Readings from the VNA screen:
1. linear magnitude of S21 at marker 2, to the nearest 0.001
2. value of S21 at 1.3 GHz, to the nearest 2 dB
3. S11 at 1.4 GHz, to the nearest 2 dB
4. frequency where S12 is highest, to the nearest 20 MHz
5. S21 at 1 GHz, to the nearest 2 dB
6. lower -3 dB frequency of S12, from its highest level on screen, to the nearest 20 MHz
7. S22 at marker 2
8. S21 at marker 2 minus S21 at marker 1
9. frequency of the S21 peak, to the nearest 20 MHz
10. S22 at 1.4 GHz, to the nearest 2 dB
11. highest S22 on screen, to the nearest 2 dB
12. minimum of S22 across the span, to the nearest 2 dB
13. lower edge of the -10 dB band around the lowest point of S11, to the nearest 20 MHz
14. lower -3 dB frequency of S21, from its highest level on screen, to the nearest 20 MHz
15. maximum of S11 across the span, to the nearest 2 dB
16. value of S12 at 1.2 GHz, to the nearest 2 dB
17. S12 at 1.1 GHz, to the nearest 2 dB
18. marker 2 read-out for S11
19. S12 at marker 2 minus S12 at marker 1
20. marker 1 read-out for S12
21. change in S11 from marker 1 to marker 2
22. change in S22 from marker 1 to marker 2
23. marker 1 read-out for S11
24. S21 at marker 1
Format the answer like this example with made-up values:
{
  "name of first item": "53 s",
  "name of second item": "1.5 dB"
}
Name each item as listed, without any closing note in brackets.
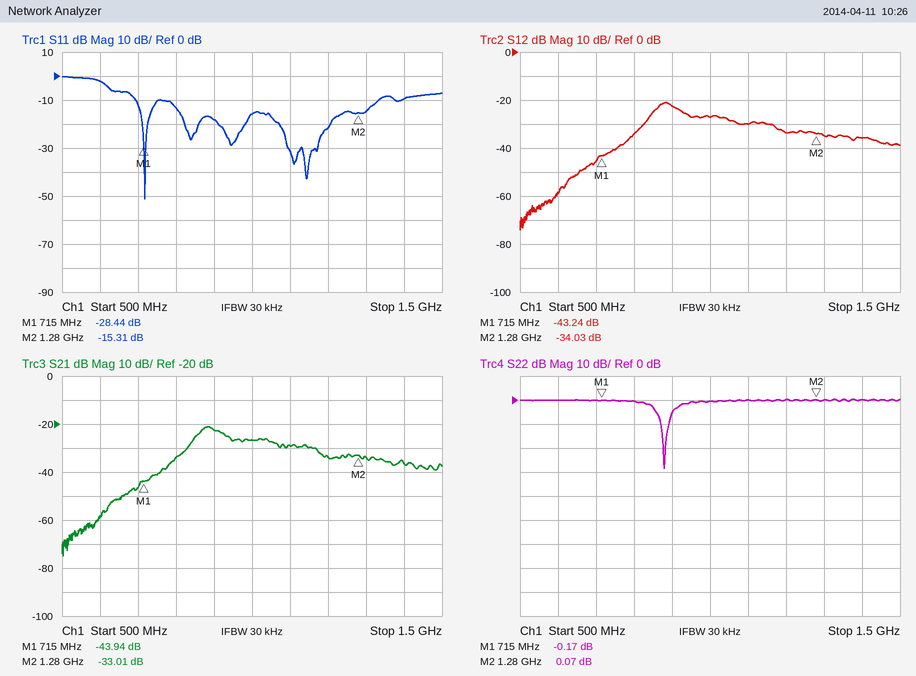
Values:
{
  "linear magnitude of S21 at marker 2, to the nearest 0.001": "0.022",
  "value of S21 at 1.3 GHz, to the nearest 2 dB": "-34 dB",
  "S11 at 1.4 GHz, to the nearest 2 dB": "-10 dB",
  "frequency where S12 is highest, to the nearest 20 MHz": "880 MHz",
  "S21 at 1 GHz, to the nearest 2 dB": "-26 dB",
  "lower -3 dB frequency of S12, from its highest level on screen, to the nearest 20 MHz": "860 MHz",
  "S22 at marker 2": "0.07 dB",
  "S21 at marker 2 minus S21 at marker 1": "10.93 dB",
  "frequency of the S21 peak, to the nearest 20 MHz": "880 MHz",
  "S22 at 1.4 GHz, to the nearest 2 dB": "0 dB",
  "highest S22 on screen, to the nearest 2 dB": "0 dB",
  "minimum of S22 across the span, to the nearest 2 dB": "-28 dB",
  "lower edge of the -10 dB band around the lowest point of S11, to the nearest 20 MHz": "700 MHz",
  "lower -3 dB frequency of S21, from its highest level on screen, to the nearest 20 MHz": "860 MHz",
  "maximum of S11 across the span, to the nearest 2 dB": "0 dB",
  "value of S12 at 1.2 GHz, to the nearest 2 dB": "-34 dB",
  "S12 at 1.1 GHz, to the nearest 2 dB": "-30 dB",
  "marker 2 read-out for S11": "-15.31 dB",
  "S12 at marker 2 minus S12 at marker 1": "9.21 dB",
  "marker 1 read-out for S12": "-43.24 dB",
  "change in S11 from marker 1 to marker 2": "13.13 dB",
  "change in S22 from marker 1 to marker 2": "0.24 dB",
  "marker 1 read-out for S11": "-28.44 dB",
  "S21 at marker 1": "-43.94 dB"
}
